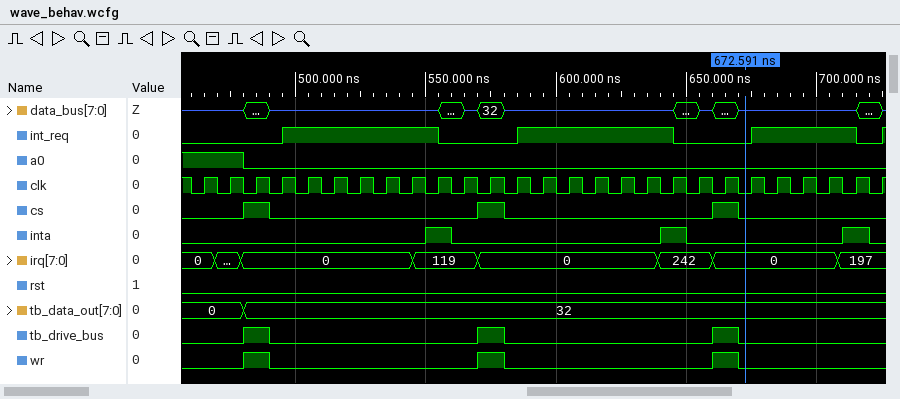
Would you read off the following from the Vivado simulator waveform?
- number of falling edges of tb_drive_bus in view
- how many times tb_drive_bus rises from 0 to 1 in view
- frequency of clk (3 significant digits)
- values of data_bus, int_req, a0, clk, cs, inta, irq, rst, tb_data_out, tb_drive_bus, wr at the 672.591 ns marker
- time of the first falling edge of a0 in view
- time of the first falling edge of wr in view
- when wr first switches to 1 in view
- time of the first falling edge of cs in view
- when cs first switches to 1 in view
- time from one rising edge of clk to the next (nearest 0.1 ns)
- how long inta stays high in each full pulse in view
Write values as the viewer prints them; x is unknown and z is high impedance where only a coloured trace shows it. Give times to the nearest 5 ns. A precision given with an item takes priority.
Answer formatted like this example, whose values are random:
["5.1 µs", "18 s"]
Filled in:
["3", "3", "100 MHz", "data_bus=z, int_req=0, a0=0, clk=0, cs=0, inta=0, irq=0, rst=0, tb_data_out=32, tb_drive_bus=0, wr=0", "480 ns", "490 ns", "480 ns", "490 ns", "480 ns", "10 ns", "10 ns, 10 ns, 10 ns"]
